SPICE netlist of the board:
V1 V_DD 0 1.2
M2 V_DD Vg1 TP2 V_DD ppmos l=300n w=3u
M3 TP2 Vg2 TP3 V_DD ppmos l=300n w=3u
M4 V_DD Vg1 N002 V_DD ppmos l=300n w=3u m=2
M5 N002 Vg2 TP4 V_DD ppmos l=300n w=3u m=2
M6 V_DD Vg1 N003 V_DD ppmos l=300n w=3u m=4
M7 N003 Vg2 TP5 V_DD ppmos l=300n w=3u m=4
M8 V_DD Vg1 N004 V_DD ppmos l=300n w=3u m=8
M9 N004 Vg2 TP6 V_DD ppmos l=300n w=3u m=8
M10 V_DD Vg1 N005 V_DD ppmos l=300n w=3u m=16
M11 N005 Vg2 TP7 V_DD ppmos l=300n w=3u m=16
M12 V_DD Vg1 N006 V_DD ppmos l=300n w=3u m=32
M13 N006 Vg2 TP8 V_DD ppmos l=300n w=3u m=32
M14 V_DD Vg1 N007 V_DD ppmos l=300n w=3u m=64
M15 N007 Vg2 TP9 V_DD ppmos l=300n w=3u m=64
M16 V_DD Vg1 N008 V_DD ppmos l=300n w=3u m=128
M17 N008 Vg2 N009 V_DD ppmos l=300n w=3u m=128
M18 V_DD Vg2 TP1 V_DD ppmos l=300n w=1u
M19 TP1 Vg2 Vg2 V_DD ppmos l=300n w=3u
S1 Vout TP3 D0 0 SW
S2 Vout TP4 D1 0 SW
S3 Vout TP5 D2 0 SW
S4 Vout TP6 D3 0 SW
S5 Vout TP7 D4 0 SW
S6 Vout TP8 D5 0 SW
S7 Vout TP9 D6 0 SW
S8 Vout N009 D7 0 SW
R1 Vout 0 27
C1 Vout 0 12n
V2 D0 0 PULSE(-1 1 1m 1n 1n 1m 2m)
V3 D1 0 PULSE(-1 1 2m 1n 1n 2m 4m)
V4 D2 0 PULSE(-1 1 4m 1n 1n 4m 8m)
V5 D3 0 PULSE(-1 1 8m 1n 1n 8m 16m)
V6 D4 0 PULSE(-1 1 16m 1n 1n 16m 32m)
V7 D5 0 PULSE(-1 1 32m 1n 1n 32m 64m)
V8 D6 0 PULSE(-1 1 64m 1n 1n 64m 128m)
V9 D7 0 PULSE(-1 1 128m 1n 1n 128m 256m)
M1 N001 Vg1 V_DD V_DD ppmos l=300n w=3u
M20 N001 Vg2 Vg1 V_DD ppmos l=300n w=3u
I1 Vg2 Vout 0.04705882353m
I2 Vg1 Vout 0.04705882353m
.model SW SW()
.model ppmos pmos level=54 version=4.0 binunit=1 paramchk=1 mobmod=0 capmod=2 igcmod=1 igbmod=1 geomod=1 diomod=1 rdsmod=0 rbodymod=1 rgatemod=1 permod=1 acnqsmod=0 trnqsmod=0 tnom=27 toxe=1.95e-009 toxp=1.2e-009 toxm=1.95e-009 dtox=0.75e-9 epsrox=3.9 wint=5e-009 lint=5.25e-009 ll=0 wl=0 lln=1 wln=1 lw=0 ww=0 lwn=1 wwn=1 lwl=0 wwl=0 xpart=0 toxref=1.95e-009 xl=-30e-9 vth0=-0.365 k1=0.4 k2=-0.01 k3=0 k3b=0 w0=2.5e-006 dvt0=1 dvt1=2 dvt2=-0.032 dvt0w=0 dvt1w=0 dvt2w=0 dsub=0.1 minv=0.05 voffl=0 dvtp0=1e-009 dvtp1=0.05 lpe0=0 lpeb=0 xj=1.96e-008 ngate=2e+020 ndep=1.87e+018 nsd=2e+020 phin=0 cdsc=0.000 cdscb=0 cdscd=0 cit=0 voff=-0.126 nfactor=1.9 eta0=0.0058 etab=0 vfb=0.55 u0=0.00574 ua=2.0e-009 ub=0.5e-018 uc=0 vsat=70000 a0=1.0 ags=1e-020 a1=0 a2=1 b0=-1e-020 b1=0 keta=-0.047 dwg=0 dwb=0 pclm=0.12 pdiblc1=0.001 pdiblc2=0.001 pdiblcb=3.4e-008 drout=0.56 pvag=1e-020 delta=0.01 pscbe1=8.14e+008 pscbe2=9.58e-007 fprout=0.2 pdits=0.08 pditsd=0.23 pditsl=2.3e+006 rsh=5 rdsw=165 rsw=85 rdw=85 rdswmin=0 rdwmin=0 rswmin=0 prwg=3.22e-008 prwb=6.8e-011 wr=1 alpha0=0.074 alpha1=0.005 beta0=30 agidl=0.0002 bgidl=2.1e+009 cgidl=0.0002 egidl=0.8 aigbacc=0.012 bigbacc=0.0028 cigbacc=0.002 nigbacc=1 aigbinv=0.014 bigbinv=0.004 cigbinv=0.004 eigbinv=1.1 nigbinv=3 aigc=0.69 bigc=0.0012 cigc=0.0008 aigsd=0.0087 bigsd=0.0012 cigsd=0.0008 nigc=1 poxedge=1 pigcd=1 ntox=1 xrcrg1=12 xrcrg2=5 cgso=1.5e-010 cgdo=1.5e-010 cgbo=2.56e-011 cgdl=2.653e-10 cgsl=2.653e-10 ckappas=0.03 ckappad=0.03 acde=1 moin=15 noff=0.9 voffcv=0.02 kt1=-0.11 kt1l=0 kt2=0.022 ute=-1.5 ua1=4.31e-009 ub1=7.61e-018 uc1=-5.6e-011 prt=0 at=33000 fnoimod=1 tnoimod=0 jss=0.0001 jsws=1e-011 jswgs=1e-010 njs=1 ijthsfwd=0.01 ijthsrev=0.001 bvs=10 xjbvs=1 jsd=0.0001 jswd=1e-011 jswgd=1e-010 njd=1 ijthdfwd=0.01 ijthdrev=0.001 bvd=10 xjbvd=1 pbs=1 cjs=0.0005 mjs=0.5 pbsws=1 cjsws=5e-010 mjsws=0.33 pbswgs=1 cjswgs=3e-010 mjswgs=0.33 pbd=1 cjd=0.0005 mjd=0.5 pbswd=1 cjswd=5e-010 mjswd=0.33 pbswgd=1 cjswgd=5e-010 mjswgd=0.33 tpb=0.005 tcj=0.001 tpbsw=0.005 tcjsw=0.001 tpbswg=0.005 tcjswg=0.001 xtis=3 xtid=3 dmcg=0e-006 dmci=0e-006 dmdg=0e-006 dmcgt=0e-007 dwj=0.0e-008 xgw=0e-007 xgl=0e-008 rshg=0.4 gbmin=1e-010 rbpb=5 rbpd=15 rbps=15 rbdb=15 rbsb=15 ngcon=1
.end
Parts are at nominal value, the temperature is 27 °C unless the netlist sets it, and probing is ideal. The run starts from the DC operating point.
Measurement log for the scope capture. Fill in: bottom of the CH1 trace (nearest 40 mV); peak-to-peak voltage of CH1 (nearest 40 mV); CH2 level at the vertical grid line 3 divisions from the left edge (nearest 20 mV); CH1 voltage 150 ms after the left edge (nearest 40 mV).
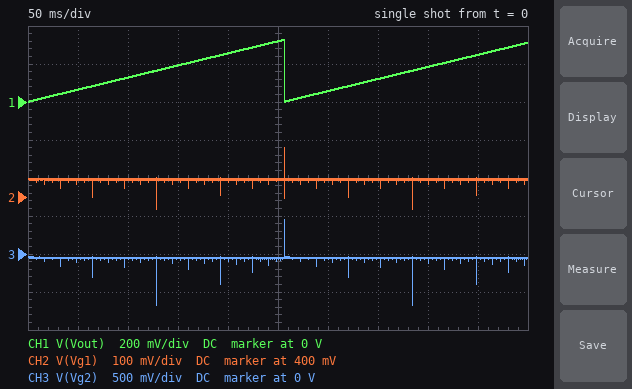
0 V
320 mV
440 mV
200 mV
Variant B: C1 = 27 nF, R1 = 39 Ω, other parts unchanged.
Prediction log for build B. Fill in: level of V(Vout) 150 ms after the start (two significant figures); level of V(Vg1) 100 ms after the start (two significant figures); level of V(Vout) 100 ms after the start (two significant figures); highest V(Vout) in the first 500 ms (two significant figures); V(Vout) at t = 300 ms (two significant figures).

280 mV
450 mV
190 mV
470 mV
83 mV
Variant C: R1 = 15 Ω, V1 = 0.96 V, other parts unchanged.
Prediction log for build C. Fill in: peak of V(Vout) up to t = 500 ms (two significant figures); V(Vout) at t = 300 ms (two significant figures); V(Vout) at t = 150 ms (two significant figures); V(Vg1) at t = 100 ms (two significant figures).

180 mV
32 mV
110 mV
210 mV
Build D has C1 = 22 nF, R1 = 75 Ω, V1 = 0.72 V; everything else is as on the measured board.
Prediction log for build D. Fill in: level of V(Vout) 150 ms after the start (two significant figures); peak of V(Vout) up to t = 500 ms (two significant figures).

410 mV
520 mV
